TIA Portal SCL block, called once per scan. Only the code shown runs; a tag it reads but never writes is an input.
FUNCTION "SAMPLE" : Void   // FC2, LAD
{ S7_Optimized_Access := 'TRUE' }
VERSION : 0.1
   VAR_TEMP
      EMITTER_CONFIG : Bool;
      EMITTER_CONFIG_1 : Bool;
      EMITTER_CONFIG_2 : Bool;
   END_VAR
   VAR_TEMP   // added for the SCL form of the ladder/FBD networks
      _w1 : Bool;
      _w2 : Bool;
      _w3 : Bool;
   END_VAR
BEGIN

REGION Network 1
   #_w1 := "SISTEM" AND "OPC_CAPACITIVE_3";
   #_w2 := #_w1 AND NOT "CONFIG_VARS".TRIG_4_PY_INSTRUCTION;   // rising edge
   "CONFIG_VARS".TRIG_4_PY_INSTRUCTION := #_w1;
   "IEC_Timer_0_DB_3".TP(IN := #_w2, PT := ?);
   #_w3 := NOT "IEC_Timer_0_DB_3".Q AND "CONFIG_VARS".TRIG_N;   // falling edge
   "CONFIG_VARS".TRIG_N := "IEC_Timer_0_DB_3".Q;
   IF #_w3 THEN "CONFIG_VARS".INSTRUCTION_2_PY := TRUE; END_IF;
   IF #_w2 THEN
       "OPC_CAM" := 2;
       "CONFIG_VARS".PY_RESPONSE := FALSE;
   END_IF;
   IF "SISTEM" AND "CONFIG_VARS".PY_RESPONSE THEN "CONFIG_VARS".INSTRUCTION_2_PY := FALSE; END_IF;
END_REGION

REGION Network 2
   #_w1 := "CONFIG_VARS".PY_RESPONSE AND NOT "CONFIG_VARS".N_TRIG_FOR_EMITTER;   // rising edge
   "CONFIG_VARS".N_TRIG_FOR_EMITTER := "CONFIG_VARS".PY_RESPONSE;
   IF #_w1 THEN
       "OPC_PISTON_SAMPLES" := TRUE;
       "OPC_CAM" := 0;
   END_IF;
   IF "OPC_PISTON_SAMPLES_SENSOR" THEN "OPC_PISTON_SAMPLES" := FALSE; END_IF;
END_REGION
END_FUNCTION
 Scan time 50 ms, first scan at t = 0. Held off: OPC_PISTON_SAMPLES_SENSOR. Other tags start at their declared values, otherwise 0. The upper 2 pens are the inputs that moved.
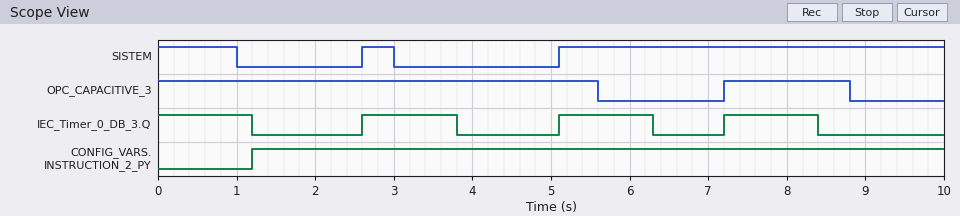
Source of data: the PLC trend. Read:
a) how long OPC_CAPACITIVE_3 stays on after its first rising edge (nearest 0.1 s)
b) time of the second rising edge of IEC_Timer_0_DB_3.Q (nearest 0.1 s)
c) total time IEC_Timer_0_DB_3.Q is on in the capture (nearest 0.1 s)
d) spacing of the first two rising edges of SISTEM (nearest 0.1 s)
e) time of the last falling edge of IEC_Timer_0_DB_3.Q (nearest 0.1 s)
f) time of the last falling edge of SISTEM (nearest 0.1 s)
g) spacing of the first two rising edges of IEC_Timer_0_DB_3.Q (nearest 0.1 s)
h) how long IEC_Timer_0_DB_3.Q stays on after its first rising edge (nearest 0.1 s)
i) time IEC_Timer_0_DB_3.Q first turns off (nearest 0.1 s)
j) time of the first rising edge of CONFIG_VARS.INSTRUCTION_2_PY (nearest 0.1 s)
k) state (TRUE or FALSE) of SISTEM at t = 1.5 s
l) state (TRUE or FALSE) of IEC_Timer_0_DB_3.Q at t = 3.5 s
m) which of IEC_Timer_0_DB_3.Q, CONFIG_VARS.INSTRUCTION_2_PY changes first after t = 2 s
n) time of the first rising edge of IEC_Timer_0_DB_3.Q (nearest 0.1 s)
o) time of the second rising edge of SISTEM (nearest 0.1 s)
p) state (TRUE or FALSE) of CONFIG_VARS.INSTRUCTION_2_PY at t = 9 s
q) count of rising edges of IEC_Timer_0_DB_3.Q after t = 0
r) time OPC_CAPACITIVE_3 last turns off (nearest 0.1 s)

1.6 s
5.1 s
4.8 s
2.5 s
8.4 s
3.0 s
2.5 s
1.2 s
1.2 s
1.2 s
FALSE
TRUE
IEC_Timer_0_DB_3.Q
2.6 s
5.1 s
TRUE
3
8.8 s
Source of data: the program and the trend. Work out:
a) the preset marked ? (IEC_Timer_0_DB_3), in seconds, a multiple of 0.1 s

1.2 s
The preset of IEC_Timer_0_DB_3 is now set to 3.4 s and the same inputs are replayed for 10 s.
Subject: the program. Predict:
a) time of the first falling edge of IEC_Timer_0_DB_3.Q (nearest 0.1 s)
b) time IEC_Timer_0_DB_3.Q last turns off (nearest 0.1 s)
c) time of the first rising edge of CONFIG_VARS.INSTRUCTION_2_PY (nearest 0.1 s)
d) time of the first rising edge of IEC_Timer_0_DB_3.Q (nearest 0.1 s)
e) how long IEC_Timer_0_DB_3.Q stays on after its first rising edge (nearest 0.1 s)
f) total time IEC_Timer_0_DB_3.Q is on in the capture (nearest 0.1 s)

3.4 s
8.5 s
3.4 s
5.1 s
3.4 s
6.8 s
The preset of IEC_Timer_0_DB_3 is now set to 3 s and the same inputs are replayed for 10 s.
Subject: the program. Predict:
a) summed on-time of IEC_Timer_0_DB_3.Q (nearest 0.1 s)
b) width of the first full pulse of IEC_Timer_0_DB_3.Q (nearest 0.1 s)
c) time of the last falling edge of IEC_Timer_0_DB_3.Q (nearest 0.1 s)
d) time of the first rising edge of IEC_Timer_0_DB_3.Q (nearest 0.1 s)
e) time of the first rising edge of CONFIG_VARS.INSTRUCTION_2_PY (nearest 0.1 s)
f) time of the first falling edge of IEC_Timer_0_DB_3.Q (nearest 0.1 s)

6.0 s
3.0 s
8.1 s
5.1 s
3.0 s
3.0 s
